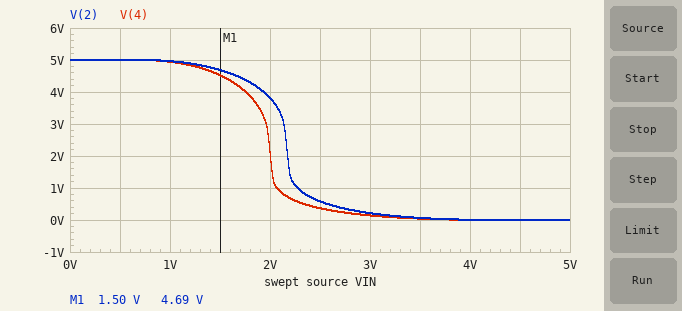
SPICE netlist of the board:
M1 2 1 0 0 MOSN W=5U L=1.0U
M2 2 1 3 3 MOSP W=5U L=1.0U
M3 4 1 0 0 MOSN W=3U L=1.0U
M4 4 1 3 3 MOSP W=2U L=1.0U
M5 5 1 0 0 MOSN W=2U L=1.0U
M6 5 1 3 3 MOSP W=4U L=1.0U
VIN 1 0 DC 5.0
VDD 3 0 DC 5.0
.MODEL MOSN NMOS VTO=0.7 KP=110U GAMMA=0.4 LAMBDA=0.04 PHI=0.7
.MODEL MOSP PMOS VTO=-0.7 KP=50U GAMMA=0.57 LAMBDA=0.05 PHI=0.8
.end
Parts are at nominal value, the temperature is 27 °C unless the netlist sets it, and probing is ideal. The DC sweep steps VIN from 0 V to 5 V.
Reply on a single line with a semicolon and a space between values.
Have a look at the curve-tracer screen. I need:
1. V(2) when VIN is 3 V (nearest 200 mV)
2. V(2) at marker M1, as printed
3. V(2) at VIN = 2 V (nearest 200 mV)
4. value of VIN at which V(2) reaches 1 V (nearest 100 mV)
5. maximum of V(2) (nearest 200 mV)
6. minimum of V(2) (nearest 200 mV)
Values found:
200 mV; 4.69 V; 3.8 V; 2.3 V; 5.0 V; 0 V
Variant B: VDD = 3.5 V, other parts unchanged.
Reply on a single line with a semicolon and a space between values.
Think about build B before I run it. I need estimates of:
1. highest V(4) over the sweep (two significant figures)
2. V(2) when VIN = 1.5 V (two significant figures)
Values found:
3.5 V; 2.6 V
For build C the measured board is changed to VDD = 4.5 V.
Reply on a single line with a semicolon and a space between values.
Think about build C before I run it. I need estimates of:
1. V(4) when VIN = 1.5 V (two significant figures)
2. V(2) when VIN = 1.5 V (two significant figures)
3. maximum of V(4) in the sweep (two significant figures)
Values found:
3.9 V; 4.1 V; 4.5 V
